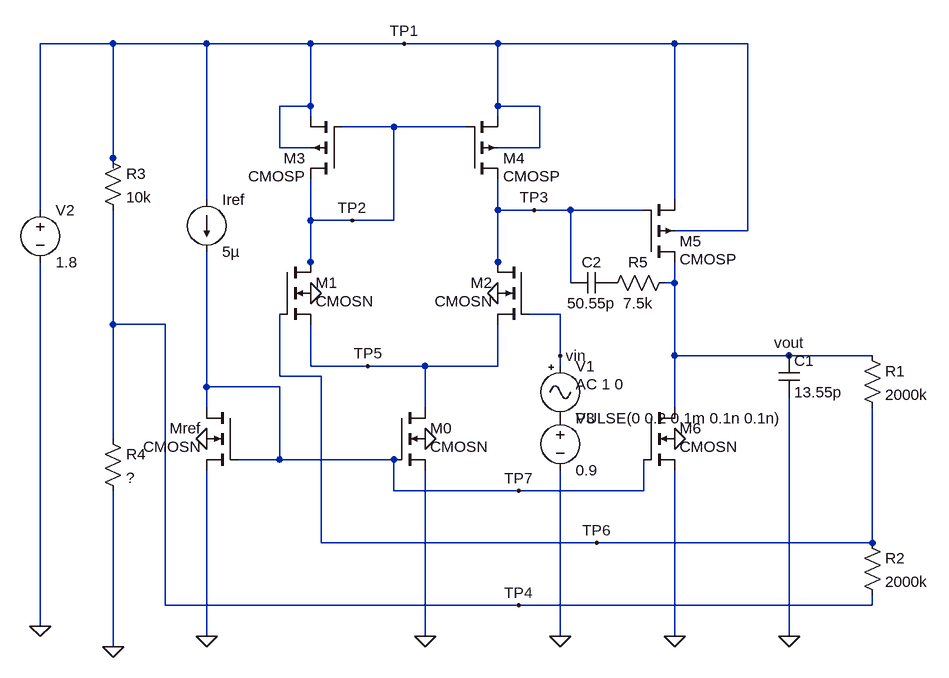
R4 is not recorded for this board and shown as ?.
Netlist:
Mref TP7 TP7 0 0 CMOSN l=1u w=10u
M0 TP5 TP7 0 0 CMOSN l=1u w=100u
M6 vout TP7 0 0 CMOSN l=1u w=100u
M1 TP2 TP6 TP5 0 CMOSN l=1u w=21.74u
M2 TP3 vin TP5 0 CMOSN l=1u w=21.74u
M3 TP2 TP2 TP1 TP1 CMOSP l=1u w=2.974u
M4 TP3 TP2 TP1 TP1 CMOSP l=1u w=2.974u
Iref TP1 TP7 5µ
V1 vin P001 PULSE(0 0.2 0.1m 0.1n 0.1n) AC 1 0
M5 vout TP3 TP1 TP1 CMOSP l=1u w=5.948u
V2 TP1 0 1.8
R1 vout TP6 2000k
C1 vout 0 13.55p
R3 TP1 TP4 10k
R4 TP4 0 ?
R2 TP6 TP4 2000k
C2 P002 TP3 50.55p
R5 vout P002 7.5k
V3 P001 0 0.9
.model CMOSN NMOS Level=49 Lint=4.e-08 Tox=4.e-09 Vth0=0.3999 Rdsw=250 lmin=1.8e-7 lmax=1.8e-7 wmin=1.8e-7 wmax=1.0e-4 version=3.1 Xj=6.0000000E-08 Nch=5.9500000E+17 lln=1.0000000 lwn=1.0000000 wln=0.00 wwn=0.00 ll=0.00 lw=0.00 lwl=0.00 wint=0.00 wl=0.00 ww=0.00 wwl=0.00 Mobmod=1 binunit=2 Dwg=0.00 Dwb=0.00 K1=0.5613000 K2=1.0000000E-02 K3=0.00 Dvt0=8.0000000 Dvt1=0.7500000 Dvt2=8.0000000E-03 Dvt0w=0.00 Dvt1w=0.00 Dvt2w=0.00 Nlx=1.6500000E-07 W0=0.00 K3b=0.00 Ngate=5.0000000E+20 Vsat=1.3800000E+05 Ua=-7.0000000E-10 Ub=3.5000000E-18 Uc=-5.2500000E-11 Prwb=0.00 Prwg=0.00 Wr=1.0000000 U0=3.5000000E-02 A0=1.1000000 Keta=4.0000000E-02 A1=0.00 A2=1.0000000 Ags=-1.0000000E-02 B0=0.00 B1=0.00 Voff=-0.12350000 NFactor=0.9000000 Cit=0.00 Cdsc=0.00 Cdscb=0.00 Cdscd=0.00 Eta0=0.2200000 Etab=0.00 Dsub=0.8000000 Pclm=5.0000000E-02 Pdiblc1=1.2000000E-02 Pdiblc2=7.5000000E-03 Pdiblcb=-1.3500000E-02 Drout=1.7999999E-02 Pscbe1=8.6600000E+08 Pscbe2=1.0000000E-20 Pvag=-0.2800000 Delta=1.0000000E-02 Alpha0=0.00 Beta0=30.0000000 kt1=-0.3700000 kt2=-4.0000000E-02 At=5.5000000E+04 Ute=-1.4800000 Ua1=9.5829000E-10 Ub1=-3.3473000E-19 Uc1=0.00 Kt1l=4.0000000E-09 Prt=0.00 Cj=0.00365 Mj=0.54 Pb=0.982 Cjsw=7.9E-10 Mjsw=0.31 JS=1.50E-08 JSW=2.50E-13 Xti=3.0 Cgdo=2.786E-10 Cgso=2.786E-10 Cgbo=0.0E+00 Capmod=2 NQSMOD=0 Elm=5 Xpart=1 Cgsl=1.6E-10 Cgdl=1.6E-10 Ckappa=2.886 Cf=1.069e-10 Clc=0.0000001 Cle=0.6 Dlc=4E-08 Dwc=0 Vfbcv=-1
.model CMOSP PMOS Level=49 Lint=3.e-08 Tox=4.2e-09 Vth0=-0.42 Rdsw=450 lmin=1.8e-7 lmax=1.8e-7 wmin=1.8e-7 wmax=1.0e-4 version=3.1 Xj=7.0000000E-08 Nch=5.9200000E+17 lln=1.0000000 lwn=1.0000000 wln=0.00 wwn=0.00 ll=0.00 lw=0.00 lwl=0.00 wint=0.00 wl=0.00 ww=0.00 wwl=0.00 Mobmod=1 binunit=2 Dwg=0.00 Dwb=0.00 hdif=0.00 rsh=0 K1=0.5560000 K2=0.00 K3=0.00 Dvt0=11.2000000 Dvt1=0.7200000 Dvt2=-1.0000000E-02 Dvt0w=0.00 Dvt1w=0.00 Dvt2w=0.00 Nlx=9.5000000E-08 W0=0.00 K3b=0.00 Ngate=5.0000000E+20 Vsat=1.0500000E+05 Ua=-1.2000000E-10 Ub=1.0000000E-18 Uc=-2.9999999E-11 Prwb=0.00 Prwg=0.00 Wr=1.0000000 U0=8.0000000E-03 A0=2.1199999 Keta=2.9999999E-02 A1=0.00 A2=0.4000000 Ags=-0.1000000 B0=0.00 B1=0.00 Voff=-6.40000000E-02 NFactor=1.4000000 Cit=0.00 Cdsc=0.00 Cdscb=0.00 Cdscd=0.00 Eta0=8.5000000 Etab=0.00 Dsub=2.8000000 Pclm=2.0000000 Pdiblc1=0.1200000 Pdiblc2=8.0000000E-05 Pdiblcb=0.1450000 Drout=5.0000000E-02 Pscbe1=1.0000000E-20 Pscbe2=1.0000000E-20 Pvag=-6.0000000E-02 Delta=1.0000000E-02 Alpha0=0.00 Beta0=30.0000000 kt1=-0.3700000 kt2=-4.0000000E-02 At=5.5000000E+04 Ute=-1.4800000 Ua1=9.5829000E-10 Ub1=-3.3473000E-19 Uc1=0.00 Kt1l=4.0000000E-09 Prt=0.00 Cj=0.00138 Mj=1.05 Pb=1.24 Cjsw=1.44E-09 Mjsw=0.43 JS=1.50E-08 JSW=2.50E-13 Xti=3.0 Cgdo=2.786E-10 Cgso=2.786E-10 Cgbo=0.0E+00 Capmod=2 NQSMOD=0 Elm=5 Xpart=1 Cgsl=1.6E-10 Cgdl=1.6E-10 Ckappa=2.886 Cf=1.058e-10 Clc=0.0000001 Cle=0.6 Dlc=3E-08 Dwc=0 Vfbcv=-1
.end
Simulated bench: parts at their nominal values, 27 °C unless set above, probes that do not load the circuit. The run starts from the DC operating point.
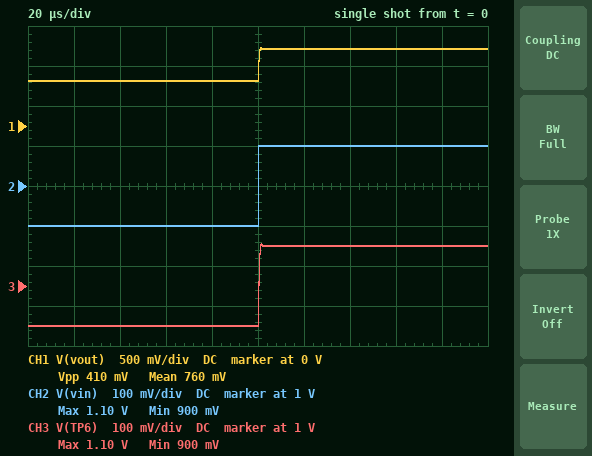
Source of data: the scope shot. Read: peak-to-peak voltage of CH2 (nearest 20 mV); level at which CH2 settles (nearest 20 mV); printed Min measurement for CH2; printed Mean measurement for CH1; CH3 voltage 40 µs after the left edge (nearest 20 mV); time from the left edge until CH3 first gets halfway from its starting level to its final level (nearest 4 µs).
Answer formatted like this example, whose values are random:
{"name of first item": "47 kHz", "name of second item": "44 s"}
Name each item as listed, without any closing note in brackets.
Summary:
{"peak-to-peak voltage of CH2": "200 mV", "level at which CH2 settles": "1.10 V", "printed Min measurement for CH2": "900 mV", "printed Mean measurement for CH1": "760 mV", "CH3 voltage 40 µs after the left edge": "900 mV", "time from the left edge until CH3 first gets halfway from its starting level to its final level": "100 µs"}
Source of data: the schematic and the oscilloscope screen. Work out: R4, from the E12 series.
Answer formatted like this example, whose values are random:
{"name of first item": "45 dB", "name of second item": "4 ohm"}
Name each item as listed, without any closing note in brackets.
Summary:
{"R4, from the E12 series": "22 kΩ"}
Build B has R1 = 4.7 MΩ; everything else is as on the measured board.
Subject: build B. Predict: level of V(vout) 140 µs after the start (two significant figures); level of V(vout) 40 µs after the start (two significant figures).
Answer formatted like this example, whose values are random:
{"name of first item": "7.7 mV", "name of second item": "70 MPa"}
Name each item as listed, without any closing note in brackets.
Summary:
{"level of V(vout) 140 µs after the start": "780 mV", "level of V(vout) 40 µs after the start": "110 mV"}
